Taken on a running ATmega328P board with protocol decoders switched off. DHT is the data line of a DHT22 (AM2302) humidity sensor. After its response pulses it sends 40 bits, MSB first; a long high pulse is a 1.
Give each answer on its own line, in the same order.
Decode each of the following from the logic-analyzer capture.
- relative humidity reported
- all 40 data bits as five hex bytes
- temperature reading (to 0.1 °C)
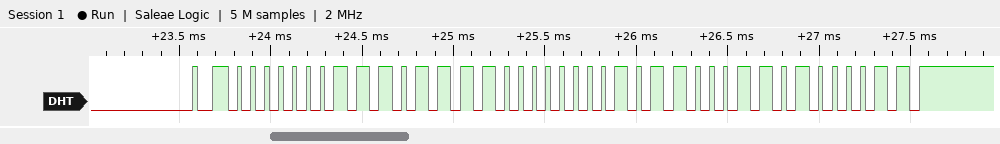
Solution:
47.8 %
01 DE 01 63 43
35.5 °C
